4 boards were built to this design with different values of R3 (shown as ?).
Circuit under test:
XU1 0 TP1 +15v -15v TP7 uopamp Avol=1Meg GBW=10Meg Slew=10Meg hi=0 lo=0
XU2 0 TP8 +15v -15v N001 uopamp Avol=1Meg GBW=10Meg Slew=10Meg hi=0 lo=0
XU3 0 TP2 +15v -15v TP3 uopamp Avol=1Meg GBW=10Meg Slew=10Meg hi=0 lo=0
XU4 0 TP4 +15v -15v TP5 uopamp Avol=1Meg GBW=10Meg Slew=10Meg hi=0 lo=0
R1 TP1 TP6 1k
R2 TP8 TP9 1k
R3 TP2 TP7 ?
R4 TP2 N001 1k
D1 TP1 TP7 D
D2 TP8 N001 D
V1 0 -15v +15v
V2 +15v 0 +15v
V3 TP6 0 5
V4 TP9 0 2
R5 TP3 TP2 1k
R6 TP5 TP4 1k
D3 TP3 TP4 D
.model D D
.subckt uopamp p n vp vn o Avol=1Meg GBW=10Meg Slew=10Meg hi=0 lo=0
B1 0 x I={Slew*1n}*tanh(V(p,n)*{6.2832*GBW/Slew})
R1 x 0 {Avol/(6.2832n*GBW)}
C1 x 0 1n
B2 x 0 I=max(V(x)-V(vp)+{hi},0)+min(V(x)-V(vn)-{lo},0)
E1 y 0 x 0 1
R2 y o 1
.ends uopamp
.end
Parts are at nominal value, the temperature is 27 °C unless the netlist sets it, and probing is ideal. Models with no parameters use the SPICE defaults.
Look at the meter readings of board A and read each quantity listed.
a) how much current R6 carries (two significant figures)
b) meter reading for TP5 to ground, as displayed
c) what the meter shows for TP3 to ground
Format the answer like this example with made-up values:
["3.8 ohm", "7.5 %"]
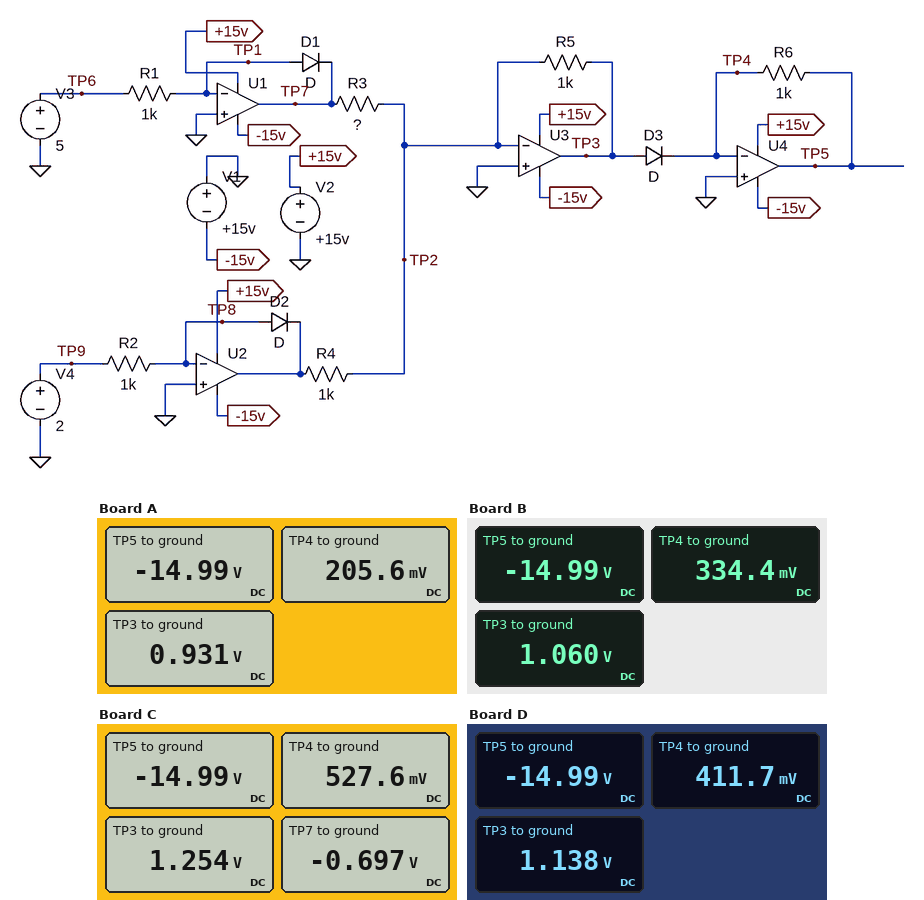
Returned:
["15 mA", "-14.99 V", "0.931 V"]
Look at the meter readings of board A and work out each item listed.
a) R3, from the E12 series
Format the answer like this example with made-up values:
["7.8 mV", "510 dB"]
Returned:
["2.7 kΩ"]
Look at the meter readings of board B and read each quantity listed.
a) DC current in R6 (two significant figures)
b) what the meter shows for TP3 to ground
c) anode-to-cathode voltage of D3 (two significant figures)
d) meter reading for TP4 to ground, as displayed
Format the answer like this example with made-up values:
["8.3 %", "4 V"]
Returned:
["15 mA", "1.060 V", "730 mV", "334.4 mV"]
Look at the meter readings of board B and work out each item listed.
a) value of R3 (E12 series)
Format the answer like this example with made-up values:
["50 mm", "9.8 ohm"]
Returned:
["1.8 kΩ"]
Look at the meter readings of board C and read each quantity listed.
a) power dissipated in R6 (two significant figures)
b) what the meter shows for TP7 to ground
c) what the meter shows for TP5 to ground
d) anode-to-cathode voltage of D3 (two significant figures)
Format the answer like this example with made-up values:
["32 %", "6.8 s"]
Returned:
["240 mW", "-0.697 V", "-14.99 V", "730 mV"]
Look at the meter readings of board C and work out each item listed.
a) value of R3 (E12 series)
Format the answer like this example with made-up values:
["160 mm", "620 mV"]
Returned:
["1.2 kΩ"]
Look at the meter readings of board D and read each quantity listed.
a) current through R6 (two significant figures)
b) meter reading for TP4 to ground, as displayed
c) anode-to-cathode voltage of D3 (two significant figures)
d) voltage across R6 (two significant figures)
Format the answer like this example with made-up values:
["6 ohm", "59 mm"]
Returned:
["15 mA", "411.7 mV", "730 mV", "15 V"]
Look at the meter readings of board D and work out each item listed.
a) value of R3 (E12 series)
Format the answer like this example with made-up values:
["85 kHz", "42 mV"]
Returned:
["1.5 kΩ"]
